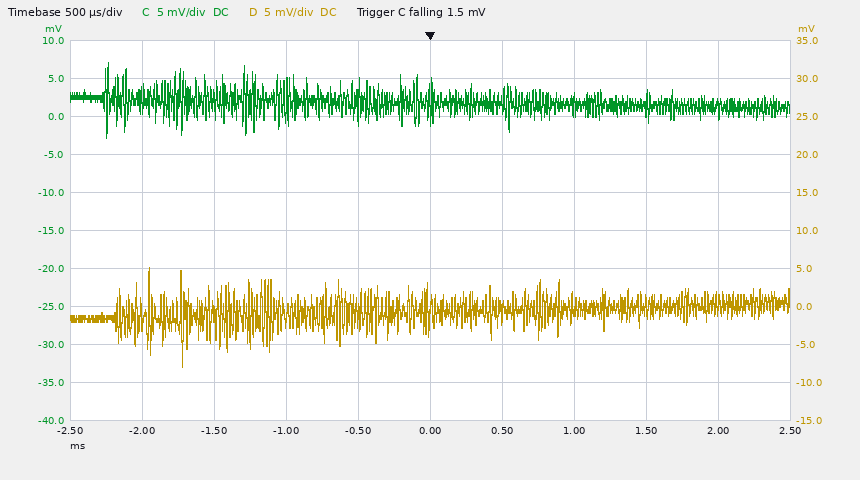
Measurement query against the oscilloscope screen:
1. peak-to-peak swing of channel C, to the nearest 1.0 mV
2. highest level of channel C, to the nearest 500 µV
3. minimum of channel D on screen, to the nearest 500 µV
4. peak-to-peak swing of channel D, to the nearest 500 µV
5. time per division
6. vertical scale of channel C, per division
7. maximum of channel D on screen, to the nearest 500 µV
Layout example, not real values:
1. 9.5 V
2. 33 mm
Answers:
1. 10.0 mV
2. 7.0 mV
3. -8.0 mV
4. 13.0 mV
5. 500 µs
6. 5 mV
7. 5.0 mV
